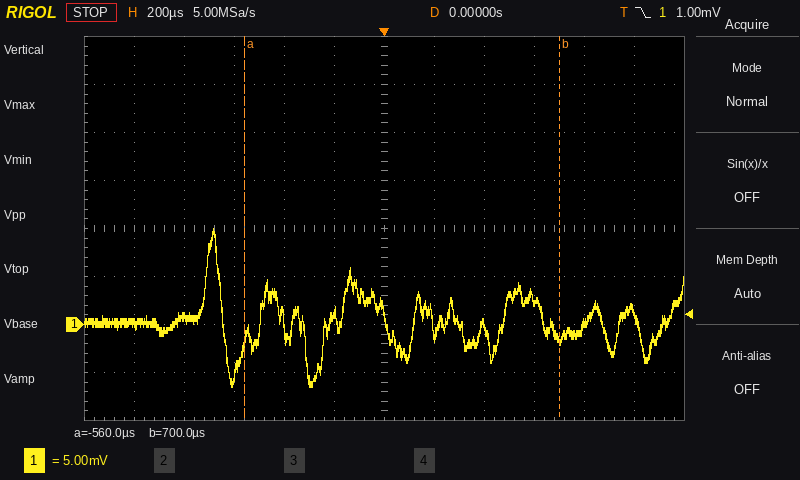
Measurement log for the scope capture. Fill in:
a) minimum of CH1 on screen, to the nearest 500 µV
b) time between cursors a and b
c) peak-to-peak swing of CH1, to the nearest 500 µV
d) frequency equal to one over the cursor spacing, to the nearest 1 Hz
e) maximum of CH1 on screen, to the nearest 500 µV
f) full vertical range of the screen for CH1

-6.5 mV
1.26 ms
16.5 mV
794 Hz
10.0 mV
40 mV
